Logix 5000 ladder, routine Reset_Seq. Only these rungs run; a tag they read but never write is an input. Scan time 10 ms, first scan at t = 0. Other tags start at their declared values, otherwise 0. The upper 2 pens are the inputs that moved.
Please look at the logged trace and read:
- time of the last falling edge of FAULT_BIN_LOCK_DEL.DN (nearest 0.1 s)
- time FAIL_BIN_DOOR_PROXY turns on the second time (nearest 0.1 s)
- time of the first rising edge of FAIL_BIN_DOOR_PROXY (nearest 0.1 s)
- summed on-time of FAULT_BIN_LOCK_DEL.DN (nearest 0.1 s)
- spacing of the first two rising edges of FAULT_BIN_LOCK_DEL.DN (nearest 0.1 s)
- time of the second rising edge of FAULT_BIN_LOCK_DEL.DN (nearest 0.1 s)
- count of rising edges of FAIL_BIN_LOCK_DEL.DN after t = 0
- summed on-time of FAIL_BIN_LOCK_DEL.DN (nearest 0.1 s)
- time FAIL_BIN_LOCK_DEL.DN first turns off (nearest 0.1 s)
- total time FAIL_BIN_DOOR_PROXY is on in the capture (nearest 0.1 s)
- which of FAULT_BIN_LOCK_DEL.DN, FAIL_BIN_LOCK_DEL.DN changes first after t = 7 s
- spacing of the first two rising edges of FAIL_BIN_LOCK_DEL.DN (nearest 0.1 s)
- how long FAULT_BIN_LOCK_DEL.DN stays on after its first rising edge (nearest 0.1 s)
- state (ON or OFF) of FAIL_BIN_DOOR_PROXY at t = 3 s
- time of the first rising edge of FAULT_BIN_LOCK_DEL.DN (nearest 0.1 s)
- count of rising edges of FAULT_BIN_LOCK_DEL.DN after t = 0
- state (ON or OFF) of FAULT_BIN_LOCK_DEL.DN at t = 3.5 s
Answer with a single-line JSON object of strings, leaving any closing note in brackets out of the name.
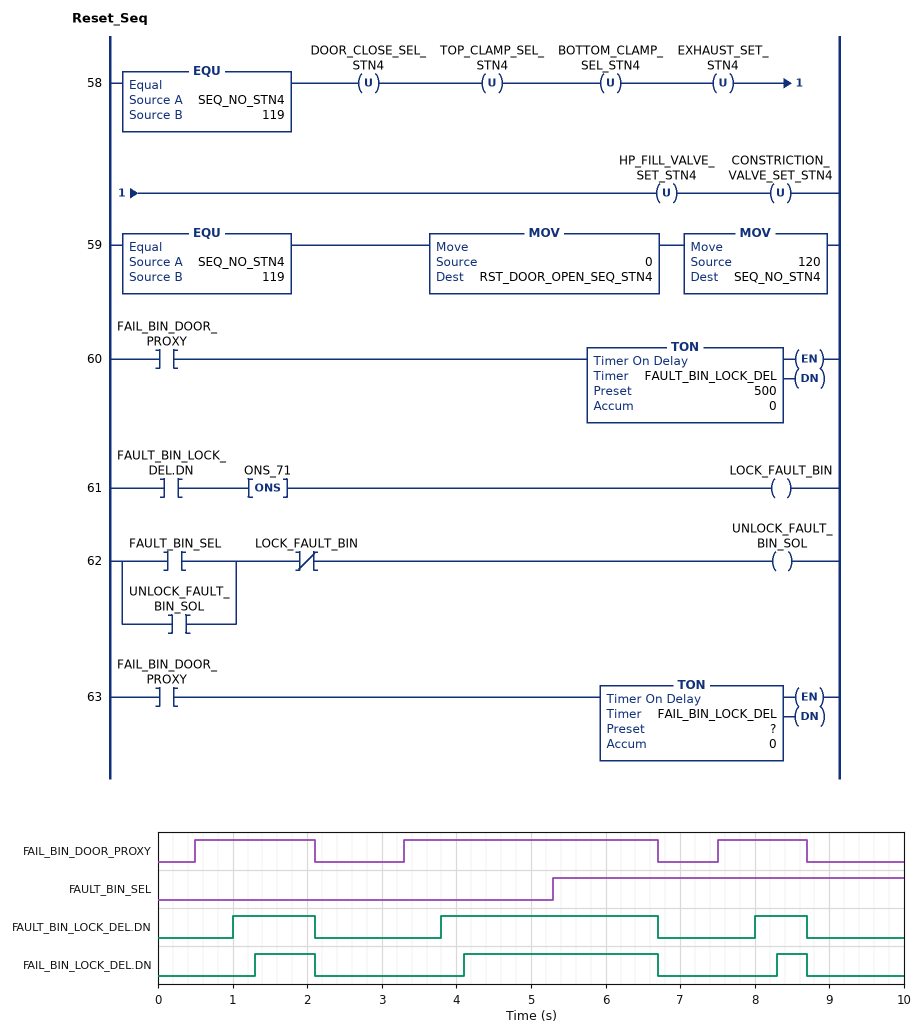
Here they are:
{"time of the last falling edge of FAULT_BIN_LOCK_DEL.DN": "8.7 s", "time FAIL_BIN_DOOR_PROXY turns on the second time": "3.3 s", "time of the first rising edge of FAIL_BIN_DOOR_PROXY": "0.5 s", "summed on-time of FAULT_BIN_LOCK_DEL.DN": "4.7 s", "spacing of the first two rising edges of FAULT_BIN_LOCK_DEL.DN": "2.8 s", "time of the second rising edge of FAULT_BIN_LOCK_DEL.DN": "3.8 s", "count of rising edges of FAIL_BIN_LOCK_DEL.DN after t = 0": "3", "summed on-time of FAIL_BIN_LOCK_DEL.DN": "3.8 s", "time FAIL_BIN_LOCK_DEL.DN first turns off": "2.1 s", "total time FAIL_BIN_DOOR_PROXY is on in the capture": "6.2 s", "which of FAULT_BIN_LOCK_DEL.DN, FAIL_BIN_LOCK_DEL.DN changes first after t = 7 s": "FAULT_BIN_LOCK_DEL.DN", "spacing of the first two rising edges of FAIL_BIN_LOCK_DEL.DN": "2.8 s", "how long FAULT_BIN_LOCK_DEL.DN stays on after its first rising edge": "1.1 s", "state (ON or OFF) of FAIL_BIN_DOOR_PROXY at t = 3 s": "OFF", "time of the first rising edge of FAULT_BIN_LOCK_DEL.DN": "1.0 s", "count of rising edges of FAULT_BIN_LOCK_DEL.DN after t = 0": "3", "state (ON or OFF) of FAULT_BIN_LOCK_DEL.DN at t = 3.5 s": "OFF"}
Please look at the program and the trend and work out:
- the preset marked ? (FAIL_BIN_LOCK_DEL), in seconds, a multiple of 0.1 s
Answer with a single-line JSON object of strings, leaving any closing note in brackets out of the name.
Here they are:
{"the preset marked ? (FAIL_BIN_LOCK_DEL), in seconds, a multiple of 0.1 s": "0.8 s"}
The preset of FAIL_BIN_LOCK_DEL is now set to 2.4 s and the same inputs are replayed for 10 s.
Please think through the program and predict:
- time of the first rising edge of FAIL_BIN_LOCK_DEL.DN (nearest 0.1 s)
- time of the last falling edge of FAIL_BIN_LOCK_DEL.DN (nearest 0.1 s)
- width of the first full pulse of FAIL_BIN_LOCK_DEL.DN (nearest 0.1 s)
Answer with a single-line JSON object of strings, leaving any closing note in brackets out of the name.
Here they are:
{"time of the first rising edge of FAIL_BIN_LOCK_DEL.DN": "5.7 s", "time of the last falling edge of FAIL_BIN_LOCK_DEL.DN": "6.7 s", "width of the first full pulse of FAIL_BIN_LOCK_DEL.DN": "1.0 s"}
